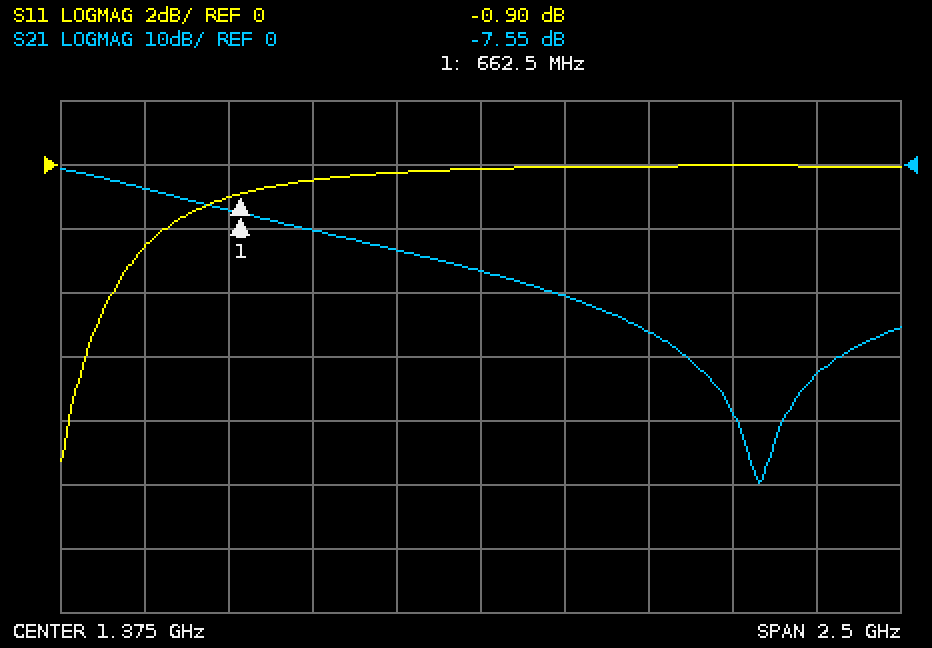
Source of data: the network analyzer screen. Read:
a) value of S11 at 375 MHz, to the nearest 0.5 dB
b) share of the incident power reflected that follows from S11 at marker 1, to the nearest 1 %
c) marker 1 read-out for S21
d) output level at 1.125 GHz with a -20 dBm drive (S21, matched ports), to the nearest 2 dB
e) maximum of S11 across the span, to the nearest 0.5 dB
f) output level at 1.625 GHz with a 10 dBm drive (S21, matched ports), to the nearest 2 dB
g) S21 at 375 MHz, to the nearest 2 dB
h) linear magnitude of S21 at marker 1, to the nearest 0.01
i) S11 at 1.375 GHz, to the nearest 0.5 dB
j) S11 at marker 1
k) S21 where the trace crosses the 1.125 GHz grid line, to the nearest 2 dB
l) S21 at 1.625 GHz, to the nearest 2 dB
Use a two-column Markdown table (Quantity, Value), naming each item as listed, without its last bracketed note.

| Quantity | Value |
|---|---|
| value of S11 at 375 MHz, to the nearest 0.5 dB | -2.5 dB |
| share of the incident power reflected that follows from S11 at marker 1, to the nearest 1 % | 81 % |
| marker 1 read-out for S21 | -7.55 dB |
| output level at 1.125 GHz with a -20 dBm drive (S21, matched ports), to the nearest 2 dB | -34 dBm |
| maximum of S11 across the span, to the nearest 0.5 dB | 0.0 dB |
| output level at 1.625 GHz with a 10 dBm drive (S21, matched ports), to the nearest 2 dB | -10 dBm |
| S21 at 375 MHz, to the nearest 2 dB | -4 dB |
| linear magnitude of S21 at marker 1, to the nearest 0.01 | 0.42 |
| S11 at 1.375 GHz, to the nearest 0.5 dB | 0.0 dB |
| S11 at marker 1 | -0.90 dB |
| S21 where the trace crosses the 1.125 GHz grid line, to the nearest 2 dB | -14 dB |
| S21 at 1.625 GHz, to the nearest 2 dB | -20 dB |
